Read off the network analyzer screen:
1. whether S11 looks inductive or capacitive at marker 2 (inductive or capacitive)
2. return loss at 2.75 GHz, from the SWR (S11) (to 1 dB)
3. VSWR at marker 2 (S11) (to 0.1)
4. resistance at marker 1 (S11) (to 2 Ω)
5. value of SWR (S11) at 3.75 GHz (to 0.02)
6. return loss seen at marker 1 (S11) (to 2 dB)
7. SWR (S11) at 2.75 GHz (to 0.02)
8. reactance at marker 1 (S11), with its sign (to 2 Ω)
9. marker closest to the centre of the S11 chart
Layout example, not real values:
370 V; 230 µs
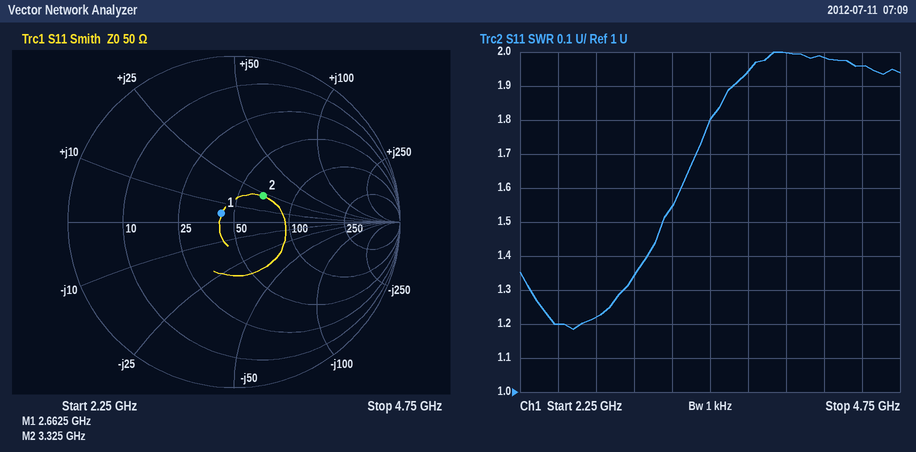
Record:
inductive; 20 dB; 1.6; 42 Ω; 1.94; 20 dB; 1.22; +4 Ω; marker 1
